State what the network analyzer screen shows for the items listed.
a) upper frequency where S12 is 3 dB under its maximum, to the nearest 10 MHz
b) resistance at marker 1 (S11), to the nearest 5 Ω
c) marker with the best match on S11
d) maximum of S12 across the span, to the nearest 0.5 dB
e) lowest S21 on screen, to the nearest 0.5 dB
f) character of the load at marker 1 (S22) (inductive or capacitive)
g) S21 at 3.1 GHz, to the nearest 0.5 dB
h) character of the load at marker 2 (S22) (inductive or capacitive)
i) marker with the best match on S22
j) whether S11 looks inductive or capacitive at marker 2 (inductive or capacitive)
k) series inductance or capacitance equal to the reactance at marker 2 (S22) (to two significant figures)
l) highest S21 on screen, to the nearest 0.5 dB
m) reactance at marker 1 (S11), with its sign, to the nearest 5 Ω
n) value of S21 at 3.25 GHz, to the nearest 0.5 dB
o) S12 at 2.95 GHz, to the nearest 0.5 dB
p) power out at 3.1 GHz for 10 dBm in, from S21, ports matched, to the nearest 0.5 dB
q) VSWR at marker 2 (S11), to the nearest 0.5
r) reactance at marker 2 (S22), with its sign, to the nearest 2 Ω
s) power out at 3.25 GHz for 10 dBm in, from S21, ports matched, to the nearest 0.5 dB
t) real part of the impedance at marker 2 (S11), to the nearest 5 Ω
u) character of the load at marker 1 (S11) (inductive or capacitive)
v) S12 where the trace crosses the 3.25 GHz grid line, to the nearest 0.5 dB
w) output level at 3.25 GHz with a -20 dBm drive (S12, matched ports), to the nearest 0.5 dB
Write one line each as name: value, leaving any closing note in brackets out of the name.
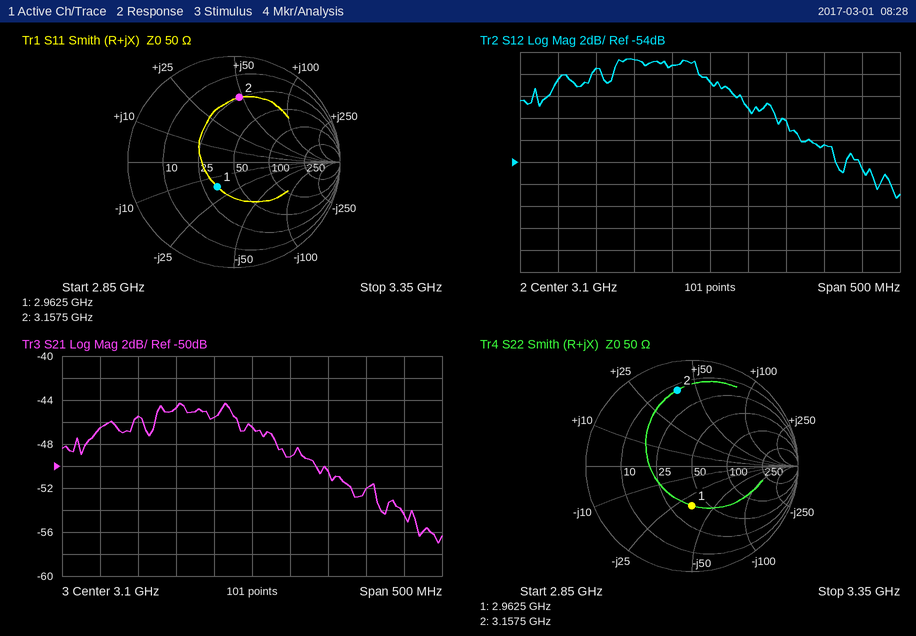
upper frequency where S12 is 3 dB under its maximum, to the nearest 10 MHz: 3.13 GHz
resistance at marker 1 (S11), to the nearest 5 Ω: 35 Ω
marker with the best match on S11: marker 1
maximum of S12 across the span, to the nearest 0.5 dB: -44.5 dB
lowest S21 on screen, to the nearest 0.5 dB: -57.0 dB
character of the load at marker 1 (S22): capacitive
S21 at 3.1 GHz, to the nearest 0.5 dB: -46.5 dB
character of the load at marker 2 (S22): inductive
marker with the best match on S22: marker 1
whether S11 looks inductive or capacitive at marker 2: inductive
series inductance or capacitance equal to the reactance at marker 2 (S22): 2.0 nH
highest S21 on screen, to the nearest 0.5 dB: -44.5 dB
reactance at marker 1 (S11), with its sign, to the nearest 5 Ω: -15 Ω
value of S21 at 3.25 GHz, to the nearest 0.5 dB: -52.0 dB
S12 at 2.95 GHz, to the nearest 0.5 dB: -45.5 dB
power out at 3.1 GHz for 10 dBm in, from S21, ports matched, to the nearest 0.5 dB: -36.5 dBm
VSWR at marker 2 (S11), to the nearest 0.5: 4.0
reactance at marker 2 (S22), with its sign, to the nearest 2 Ω: +40 Ω
power out at 3.25 GHz for 10 dBm in, from S21, ports matched, to the nearest 0.5 dB: -42.0 dBm
real part of the impedance at marker 2 (S11), to the nearest 5 Ω: 25 Ω
character of the load at marker 1 (S11): capacitive
S12 where the trace crosses the 3.25 GHz grid line, to the nearest 0.5 dB: -52.5 dB
output level at 3.25 GHz with a -20 dBm drive (S12, matched ports), to the nearest 0.5 dB: -72.5 dBm
